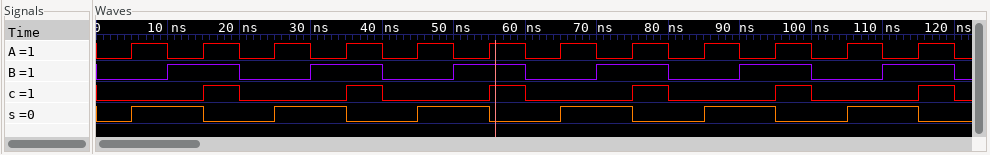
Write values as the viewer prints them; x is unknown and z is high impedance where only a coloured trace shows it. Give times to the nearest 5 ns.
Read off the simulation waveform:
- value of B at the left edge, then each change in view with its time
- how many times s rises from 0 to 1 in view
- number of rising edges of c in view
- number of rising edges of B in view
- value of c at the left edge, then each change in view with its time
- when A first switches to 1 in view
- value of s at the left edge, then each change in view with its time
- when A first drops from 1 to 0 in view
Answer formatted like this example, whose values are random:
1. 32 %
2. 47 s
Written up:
1. 0, 1 at 10 ns, 0 at 20 ns, 1 at 30 ns, 0 at 40 ns, 1 at 50 ns, 0 at 60 ns, 1 at 70 ns, 0 at 80 ns, 1 at 90 ns, 0 at 100 ns, 1 at 110 ns, 0 at 120 ns
2. 6
3. 6
4. 6
5. 0, 1 at 15 ns, 0 at 20 ns, 1 at 35 ns, 0 at 40 ns, 1 at 55 ns, 0 at 60 ns, 1 at 75 ns, 0 at 80 ns, 1 at 95 ns, 0 at 100 ns, 1 at 115 ns, 0 at 120 ns
6. 5 ns
7. 0, 1 at 5 ns, 0 at 15 ns, 1 at 25 ns, 0 at 35 ns, 1 at 45 ns, 0 at 55 ns, 1 at 65 ns, 0 at 75 ns, 1 at 85 ns, 0 at 95 ns, 1 at 105 ns, 0 at 115 ns
8. 10 ns
